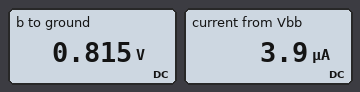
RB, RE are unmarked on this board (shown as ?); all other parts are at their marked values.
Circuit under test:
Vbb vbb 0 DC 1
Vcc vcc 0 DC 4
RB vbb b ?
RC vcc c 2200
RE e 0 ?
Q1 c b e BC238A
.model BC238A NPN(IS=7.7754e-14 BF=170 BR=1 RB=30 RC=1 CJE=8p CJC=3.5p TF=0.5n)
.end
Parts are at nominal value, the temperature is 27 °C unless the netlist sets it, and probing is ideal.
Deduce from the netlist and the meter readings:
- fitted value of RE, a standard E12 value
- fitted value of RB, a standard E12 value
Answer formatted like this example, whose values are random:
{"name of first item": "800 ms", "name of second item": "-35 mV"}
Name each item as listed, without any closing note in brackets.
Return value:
{"fitted value of RE, a standard E12 value": "330 Ω", "fitted value of RB, a standard E12 value": "47 kΩ"}
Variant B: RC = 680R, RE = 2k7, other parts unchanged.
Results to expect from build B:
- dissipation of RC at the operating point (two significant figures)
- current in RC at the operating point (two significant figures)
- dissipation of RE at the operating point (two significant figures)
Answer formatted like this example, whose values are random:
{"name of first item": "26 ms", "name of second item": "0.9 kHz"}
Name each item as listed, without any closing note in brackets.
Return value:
{"dissipation of RC at the operating point": "15 µW", "current in RC at the operating point": "150 µA", "dissipation of RE at the operating point": "61 µW"}
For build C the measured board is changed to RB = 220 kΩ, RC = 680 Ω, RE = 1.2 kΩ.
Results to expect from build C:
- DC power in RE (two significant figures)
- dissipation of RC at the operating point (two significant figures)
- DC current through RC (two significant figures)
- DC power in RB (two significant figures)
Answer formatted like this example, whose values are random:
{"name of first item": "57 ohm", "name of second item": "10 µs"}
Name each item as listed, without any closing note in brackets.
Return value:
{"DC power in RE": "38 µW", "dissipation of RC at the operating point": "21 µW", "DC current through RC": "180 µA", "DC power in RB": "240 nW"}
